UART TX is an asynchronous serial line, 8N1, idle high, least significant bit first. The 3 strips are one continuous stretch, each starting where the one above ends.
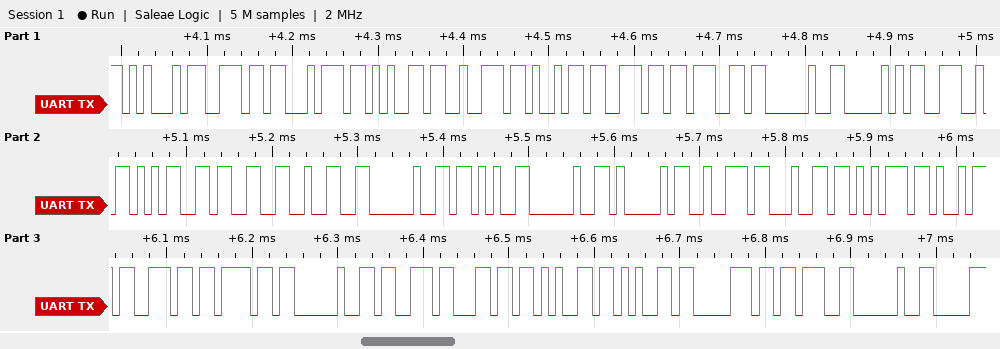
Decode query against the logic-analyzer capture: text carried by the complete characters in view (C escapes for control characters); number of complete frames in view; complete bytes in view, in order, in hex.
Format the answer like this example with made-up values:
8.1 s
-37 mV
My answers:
"Entering PN532 + Arduino sleep; "
32
0x45 0x6E 0x74 0x65 0x72 0x69 0x6E 0x67 0x20 0x50 0x4E 0x35 0x33 0x32 0x20 0x2B 0x20 0x41 0x72 0x64 0x75 0x69 0x6E 0x6F 0x20 0x73 0x6C 0x65 0x65 0x70 0x3B 0x20
